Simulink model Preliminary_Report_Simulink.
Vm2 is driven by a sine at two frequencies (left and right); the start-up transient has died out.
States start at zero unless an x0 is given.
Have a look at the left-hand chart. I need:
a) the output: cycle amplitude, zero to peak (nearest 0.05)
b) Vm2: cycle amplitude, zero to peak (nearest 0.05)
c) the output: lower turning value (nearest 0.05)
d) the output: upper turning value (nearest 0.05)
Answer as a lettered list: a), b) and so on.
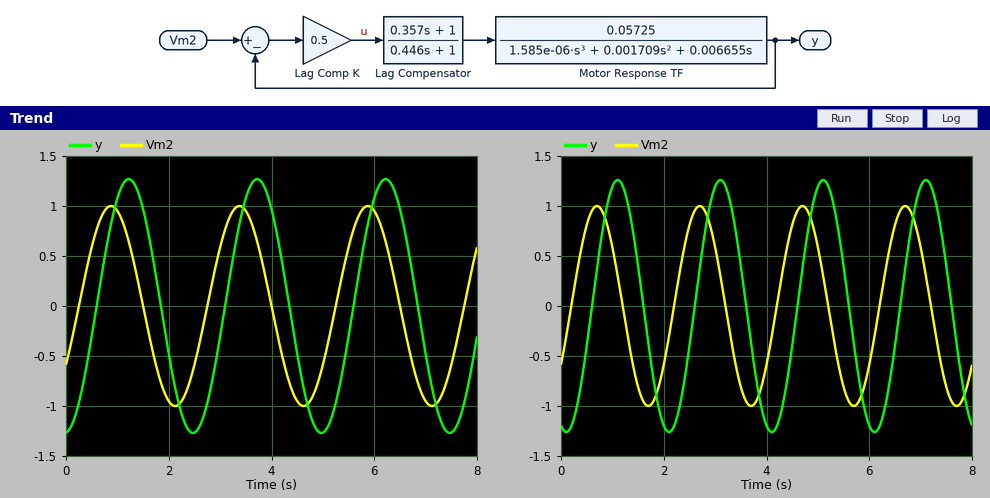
a) 1.25
b) 1.00
c) -1.25
d) 1.25
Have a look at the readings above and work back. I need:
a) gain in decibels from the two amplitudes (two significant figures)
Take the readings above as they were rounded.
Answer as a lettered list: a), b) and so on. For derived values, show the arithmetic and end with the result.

a) 20 log10(1.25 / 1) = 1.9 dB
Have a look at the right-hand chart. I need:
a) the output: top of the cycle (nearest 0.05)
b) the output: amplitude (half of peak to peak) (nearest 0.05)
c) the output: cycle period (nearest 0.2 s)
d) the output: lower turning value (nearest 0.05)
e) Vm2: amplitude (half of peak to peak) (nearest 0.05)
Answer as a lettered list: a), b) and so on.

a) 1.25
b) 1.25
c) 2.0 s
d) -1.25
e) 1.00
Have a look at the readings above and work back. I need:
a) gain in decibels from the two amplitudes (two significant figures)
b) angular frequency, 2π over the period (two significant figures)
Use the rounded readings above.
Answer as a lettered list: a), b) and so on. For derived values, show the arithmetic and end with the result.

a) 20 log10(1.25 / 1) = 1.9 dB
b) 2π / 2 = 3.1 rad/s
